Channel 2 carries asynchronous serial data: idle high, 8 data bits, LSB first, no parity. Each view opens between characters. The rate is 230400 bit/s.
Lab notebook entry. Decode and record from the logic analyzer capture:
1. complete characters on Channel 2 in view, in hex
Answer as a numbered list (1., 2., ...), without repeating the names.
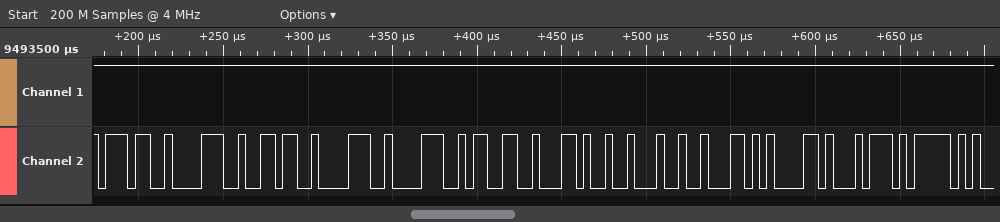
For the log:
1. 37, 38, 36, 38, 38, 33, 2C, 22, 62, 61, 74, 5F
